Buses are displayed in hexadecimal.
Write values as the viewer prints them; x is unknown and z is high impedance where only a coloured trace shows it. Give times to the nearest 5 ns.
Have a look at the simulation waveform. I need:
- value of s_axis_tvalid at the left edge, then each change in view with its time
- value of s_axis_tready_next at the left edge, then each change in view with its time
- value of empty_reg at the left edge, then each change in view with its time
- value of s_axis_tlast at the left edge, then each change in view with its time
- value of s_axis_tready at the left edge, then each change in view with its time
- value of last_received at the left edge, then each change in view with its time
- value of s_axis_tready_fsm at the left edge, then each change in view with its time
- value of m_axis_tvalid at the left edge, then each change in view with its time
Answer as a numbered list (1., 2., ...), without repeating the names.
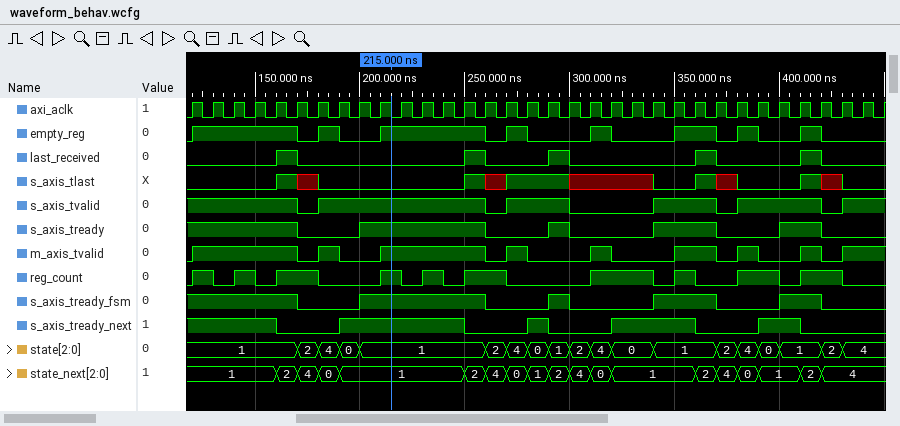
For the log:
1. 1, 0 at 170 ns, 1 at 180 ns, 0 at 260 ns, 1 at 270 ns, 0 at 300 ns, 1 at 340 ns, 0 at 370 ns, 1 at 380 ns, 0 at 420 ns, 1 at 430 ns
2. 1, 0 at 160 ns, 1 at 190 ns, 0 at 250 ns, 1 at 280 ns, 0 at 290 ns, 1 at 320 ns, 0 at 360 ns, 1 at 390 ns, 0 at 410 ns
3. 0, 1 at 120 ns, 0 at 170 ns, 1 at 180 ns, 0 at 190 ns, 1 at 210 ns, 0 at 260 ns, 1 at 270 ns, 0 at 280 ns, 1 at 310 ns, 0 at 320 ns, 1 at 350 ns, 0 at 370 ns, 1 at 380 ns, 0 at 390 ns, 1 at 410 ns, 0 at 420 ns
4. 0, 1 at 160 ns, x at 170 ns, 0 at 180 ns, 1 at 250 ns, x at 260 ns, 1 at 270 ns, x at 300 ns, 0 at 340 ns, 1 at 360 ns, x at 370 ns, 0 at 380 ns, 1 at 410 ns, x at 420 ns, 0 at 430 ns
5. 1, 0 at 170 ns, 1 at 200 ns, 0 at 260 ns, 1 at 290 ns, 0 at 300 ns, 1 at 340 ns, 0 at 370 ns, 1 at 400 ns, 0 at 420 ns
6. 0, 1 at 160 ns, 0 at 170 ns, 1 at 250 ns, 0 at 260 ns, 1 at 290 ns, 0 at 300 ns, 1 at 360 ns, 0 at 370 ns, 1 at 410 ns, 0 at 420 ns
7. 1, 0 at 170 ns, 1 at 200 ns, 0 at 260 ns, 1 at 290 ns, 0 at 300 ns, 1 at 340 ns, 0 at 370 ns, 1 at 400 ns, 0 at 420 ns
8. 0, 1 at 120 ns, 0 at 170 ns, 1 at 180 ns, 0 at 190 ns, 1 at 210 ns, 0 at 260 ns, 1 at 270 ns, 0 at 280 ns, 1 at 310 ns, 0 at 320 ns, 1 at 350 ns, 0 at 370 ns, 1 at 380 ns, 0 at 390 ns, 1 at 410 ns, 0 at 420 ns, 1 at 430 ns
